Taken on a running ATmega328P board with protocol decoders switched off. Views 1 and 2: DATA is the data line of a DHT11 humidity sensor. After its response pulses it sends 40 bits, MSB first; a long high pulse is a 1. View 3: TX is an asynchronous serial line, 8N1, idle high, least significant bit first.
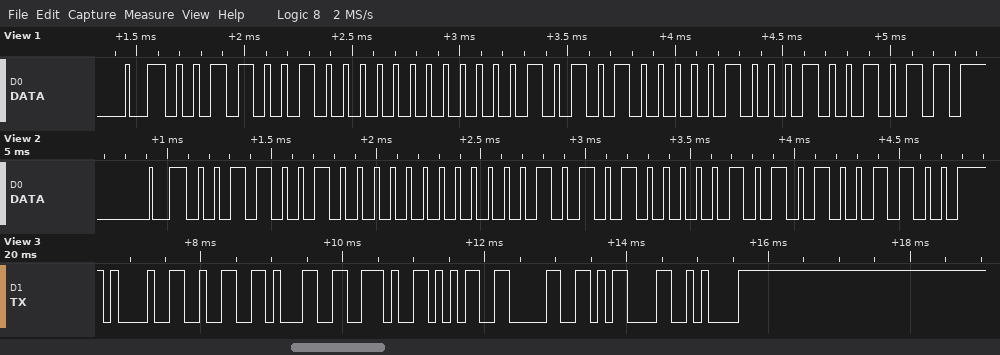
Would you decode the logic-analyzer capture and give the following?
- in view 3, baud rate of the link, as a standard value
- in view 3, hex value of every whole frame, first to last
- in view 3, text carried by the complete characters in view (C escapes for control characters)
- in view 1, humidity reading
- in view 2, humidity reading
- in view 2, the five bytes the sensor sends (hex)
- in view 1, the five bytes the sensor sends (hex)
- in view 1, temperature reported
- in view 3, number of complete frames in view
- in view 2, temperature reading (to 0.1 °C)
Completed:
9600 baud
21 32 31 2E 35 30 0D 0A
"!21.50\r\n"
50 %
50 %
32 00 15 05 4C
32 00 15 04 4B
21.4 °C
8
21.5 °C
